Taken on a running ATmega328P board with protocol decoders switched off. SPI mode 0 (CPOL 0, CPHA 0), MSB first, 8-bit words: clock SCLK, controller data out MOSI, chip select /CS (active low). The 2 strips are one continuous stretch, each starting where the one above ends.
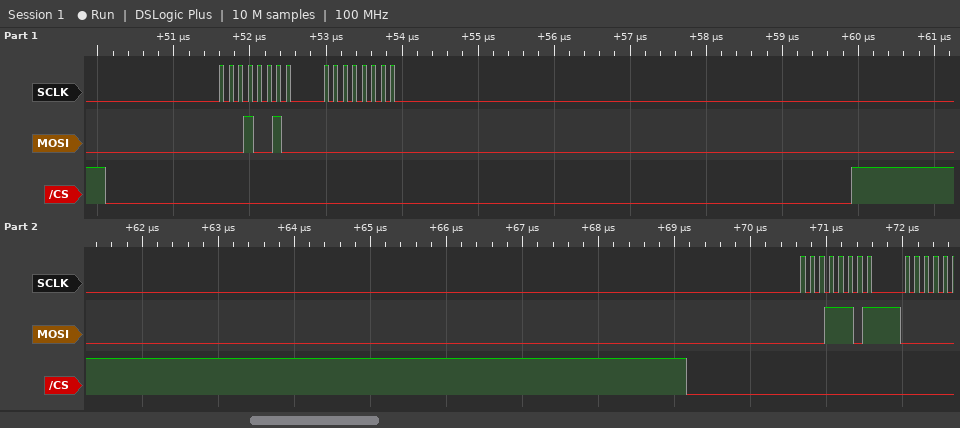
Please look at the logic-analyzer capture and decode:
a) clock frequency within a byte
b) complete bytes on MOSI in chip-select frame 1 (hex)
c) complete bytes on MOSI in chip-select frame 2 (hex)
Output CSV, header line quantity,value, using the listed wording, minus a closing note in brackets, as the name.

quantity,value
clock frequency within a byte,8 MHz
complete bytes on MOSI in chip-select frame 1,12 00
complete bytes on MOSI in chip-select frame 2,1D
